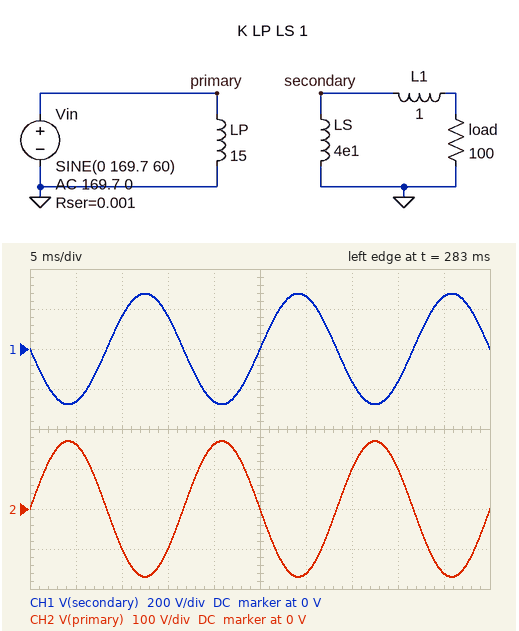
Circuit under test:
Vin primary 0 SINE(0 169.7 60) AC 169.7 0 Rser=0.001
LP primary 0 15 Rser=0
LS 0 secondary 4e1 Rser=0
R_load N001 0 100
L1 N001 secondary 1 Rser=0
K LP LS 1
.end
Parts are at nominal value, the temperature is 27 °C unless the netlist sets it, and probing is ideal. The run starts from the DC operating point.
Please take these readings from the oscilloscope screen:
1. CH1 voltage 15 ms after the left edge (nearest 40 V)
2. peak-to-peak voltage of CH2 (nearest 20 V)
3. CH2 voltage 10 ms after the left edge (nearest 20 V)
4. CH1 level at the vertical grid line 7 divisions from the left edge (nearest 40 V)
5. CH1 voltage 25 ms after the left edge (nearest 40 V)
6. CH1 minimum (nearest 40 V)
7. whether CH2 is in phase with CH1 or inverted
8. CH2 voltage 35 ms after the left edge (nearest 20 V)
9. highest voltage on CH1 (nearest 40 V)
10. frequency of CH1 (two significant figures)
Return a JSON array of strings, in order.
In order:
["160 V", "340 V", "-100 V", "-160 V", "0 V", "-280 V", "inverted", "100 V", "280 V", "60 Hz"]
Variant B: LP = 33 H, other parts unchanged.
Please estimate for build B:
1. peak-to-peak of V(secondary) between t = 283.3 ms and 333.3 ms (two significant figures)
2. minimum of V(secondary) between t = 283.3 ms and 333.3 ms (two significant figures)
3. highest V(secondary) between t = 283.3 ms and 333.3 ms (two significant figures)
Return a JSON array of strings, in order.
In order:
["370 V", "-190 V", "190 V"]
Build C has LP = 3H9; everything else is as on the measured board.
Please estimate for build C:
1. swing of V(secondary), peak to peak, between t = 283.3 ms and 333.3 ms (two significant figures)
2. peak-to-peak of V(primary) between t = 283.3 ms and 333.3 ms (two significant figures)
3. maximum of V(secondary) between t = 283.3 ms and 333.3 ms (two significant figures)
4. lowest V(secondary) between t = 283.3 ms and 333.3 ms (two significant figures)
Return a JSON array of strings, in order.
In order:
["1.1 kV", "340 V", "540 V", "-540 V"]
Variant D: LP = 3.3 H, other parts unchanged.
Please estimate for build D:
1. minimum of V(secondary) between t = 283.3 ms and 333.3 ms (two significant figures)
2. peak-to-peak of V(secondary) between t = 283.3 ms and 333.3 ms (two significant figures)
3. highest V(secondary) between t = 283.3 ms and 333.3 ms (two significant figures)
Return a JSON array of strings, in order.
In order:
["-590 V", "1.2 kV", "590 V"]
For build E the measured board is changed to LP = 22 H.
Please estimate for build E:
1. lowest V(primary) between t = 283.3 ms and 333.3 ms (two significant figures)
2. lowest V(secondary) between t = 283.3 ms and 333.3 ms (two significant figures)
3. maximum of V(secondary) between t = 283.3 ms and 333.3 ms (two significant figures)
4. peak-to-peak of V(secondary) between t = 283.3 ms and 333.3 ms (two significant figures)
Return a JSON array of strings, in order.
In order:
["-170 V", "-230 V", "230 V", "460 V"]
